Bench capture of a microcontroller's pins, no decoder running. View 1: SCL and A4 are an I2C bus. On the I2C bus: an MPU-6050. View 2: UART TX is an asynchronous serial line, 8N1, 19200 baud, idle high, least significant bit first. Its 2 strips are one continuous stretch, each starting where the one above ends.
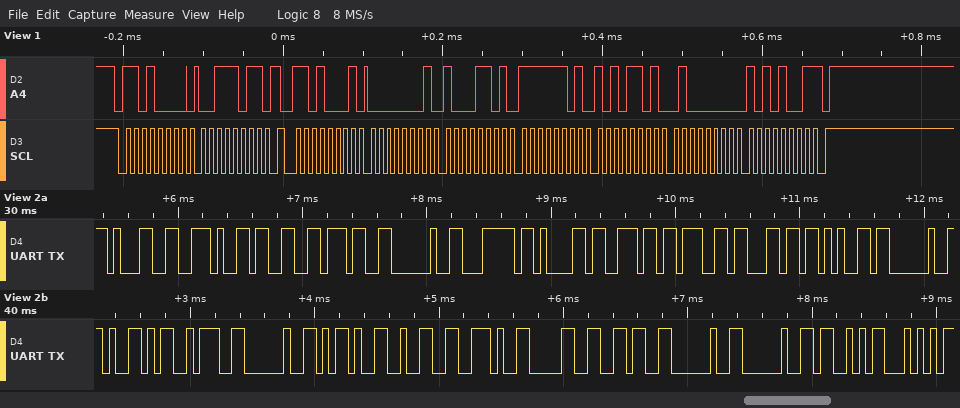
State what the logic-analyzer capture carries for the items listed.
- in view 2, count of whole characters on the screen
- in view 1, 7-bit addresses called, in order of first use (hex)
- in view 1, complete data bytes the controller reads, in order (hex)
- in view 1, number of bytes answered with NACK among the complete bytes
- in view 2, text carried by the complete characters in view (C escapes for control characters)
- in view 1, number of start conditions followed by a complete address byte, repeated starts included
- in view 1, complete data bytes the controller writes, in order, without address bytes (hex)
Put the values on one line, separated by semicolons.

24; 0x68; 01 8D FD AD 40 A9; 1; "1.37 |angle Y: -2.06  ST"; 2; 3B
